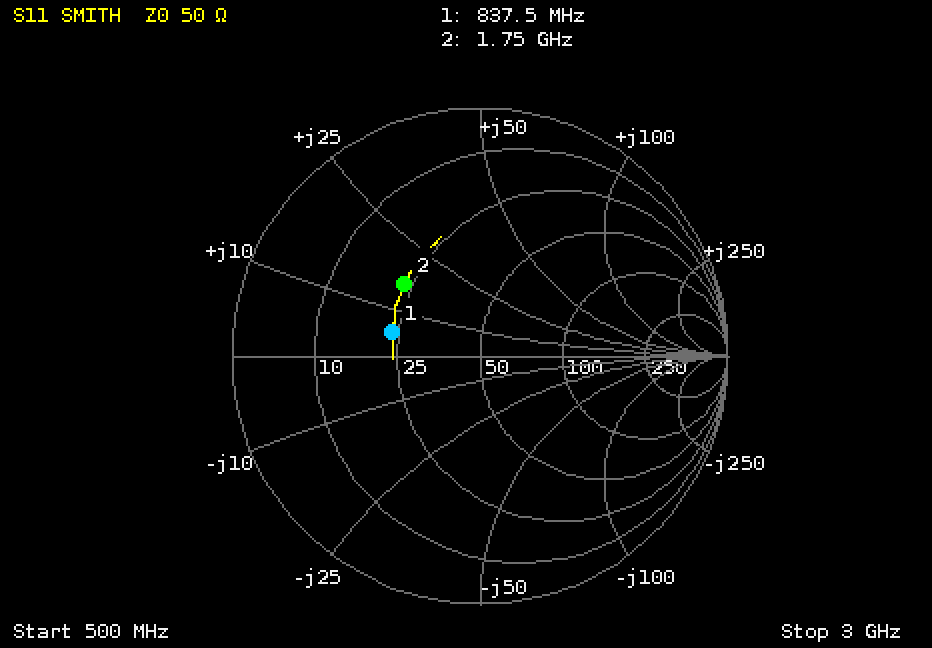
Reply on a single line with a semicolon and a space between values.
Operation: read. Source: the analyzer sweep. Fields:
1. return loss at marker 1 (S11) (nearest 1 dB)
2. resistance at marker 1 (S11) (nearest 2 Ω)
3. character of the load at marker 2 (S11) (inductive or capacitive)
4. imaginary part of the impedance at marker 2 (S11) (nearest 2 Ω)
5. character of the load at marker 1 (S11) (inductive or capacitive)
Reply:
9 dB; 24 Ω; inductive; +16 Ω; inductive
